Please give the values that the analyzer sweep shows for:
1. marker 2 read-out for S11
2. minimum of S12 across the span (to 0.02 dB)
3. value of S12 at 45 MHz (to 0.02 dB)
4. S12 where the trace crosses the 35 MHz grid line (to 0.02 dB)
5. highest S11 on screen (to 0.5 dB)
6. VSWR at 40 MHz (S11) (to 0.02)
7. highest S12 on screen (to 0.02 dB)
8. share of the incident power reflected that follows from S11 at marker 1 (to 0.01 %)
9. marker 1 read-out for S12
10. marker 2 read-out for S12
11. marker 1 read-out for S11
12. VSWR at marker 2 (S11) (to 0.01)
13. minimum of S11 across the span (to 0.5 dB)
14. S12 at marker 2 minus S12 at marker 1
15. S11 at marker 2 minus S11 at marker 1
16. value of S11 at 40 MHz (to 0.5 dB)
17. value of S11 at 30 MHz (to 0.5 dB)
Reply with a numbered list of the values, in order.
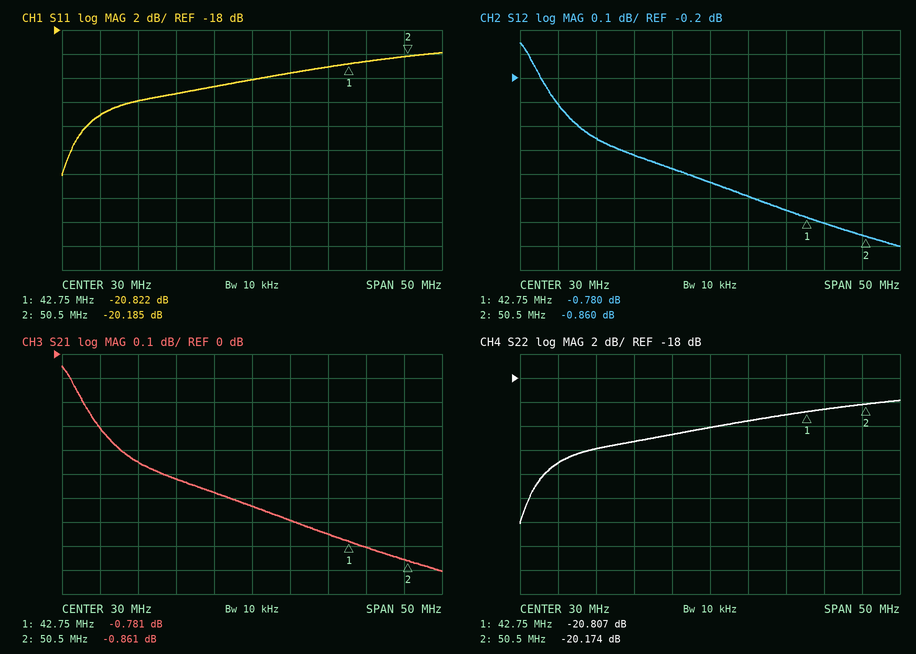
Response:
1. -20.185 dB
2. -0.90 dB
3. -0.80 dB
4. -0.70 dB
5. -20.0 dB
6. 1.20
7. -0.06 dB
8. 0.83 %
9. -0.780 dB
10. -0.860 dB
11. -20.822 dB
12. 1.22
13. -30.0 dB
14. -0.080 dB
15. 0.637 dB
16. -21.0 dB
17. -22.0 dB
